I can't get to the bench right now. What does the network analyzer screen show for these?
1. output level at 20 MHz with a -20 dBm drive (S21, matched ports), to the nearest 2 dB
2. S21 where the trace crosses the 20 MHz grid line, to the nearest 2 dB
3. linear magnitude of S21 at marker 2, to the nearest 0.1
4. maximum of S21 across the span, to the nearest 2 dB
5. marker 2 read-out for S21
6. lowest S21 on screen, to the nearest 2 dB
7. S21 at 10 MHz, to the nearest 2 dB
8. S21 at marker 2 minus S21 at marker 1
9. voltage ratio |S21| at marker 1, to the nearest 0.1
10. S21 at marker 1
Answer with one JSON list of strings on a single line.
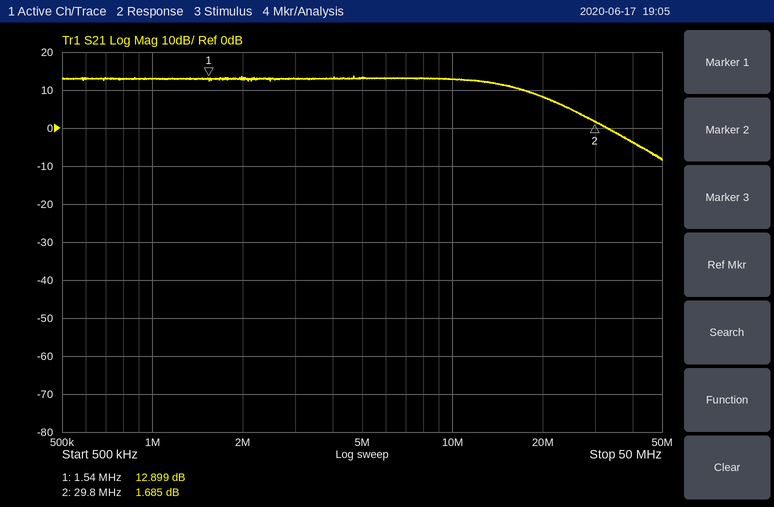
["-12 dBm", "8 dB", "1.2", "14 dB", "1.685 dB", "-8 dB", "12 dB", "-11.214 dB", "4.4", "12.899 dB"]
